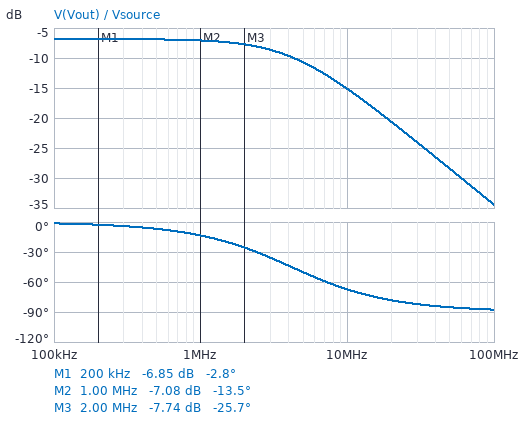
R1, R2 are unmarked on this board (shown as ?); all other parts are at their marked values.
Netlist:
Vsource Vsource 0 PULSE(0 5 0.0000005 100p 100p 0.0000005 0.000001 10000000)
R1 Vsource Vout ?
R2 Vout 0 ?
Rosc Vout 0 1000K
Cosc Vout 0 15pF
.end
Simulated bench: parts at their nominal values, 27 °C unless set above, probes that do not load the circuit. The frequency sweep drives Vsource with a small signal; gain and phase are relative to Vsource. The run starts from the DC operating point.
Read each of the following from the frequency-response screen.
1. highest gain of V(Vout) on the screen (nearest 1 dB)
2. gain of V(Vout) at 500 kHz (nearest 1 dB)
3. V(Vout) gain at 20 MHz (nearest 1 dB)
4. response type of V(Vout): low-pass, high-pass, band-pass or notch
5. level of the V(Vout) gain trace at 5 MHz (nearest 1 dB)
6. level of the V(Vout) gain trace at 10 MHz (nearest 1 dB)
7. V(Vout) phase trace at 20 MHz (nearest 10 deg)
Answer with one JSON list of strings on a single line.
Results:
["-7 dB", "-7 dB", "-21 dB", "low-pass", "-11 dB", "-15 dB", "-80 deg"]
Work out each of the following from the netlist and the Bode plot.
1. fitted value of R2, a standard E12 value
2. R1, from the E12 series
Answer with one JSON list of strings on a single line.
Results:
["4.7 kΩ", "5.6 kΩ"]
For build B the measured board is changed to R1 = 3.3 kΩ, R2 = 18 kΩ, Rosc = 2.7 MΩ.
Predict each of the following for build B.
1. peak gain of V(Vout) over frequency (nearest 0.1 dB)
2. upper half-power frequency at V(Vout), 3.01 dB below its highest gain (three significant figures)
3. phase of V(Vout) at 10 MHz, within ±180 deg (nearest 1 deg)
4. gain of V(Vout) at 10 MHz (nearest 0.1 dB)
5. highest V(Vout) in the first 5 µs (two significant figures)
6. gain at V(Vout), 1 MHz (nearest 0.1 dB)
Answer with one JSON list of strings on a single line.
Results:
["-1.5 dB", "3.81 MHz", "-69 deg", "-10.4 dB", "4.2 V", "-1.8 dB"]
